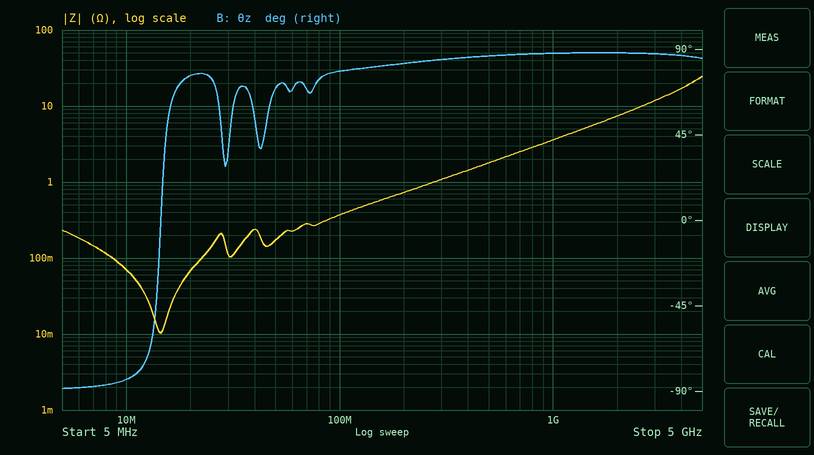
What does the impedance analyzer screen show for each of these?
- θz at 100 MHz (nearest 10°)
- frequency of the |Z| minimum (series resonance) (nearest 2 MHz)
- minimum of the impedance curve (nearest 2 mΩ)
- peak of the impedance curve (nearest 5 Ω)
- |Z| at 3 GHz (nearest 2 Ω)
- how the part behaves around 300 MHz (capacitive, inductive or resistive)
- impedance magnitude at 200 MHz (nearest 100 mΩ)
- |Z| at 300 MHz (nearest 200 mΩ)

80°
14 MHz
10 mΩ
25 Ω
12 Ω
inductive
700 mΩ
1.0 Ω
